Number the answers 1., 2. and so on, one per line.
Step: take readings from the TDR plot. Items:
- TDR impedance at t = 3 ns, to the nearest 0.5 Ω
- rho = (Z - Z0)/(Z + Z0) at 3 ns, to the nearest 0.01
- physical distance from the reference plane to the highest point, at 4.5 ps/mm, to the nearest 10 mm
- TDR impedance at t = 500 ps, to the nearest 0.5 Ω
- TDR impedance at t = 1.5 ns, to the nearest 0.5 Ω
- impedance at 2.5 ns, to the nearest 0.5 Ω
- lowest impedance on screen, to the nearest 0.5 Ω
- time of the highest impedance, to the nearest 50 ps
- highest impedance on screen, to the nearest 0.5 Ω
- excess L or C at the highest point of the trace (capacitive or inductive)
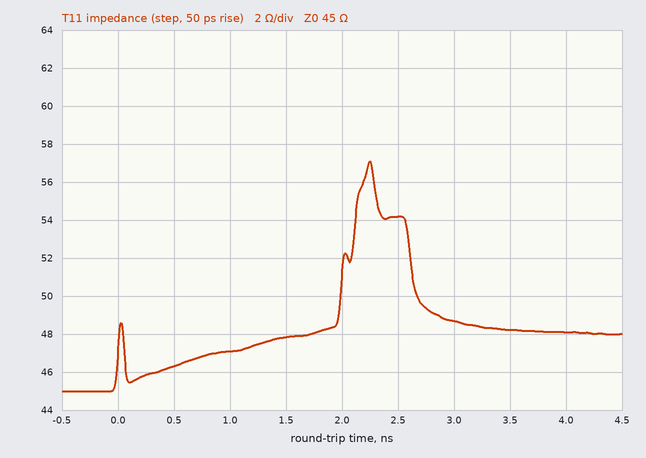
1. 48.5 Ω
2. +0.04
3. 250 mm
4. 46.5 Ω
5. 48.0 Ω
6. 54.0 Ω
7. 45.0 Ω
8. 2.25 ns
9. 57.0 Ω
10. inductive
